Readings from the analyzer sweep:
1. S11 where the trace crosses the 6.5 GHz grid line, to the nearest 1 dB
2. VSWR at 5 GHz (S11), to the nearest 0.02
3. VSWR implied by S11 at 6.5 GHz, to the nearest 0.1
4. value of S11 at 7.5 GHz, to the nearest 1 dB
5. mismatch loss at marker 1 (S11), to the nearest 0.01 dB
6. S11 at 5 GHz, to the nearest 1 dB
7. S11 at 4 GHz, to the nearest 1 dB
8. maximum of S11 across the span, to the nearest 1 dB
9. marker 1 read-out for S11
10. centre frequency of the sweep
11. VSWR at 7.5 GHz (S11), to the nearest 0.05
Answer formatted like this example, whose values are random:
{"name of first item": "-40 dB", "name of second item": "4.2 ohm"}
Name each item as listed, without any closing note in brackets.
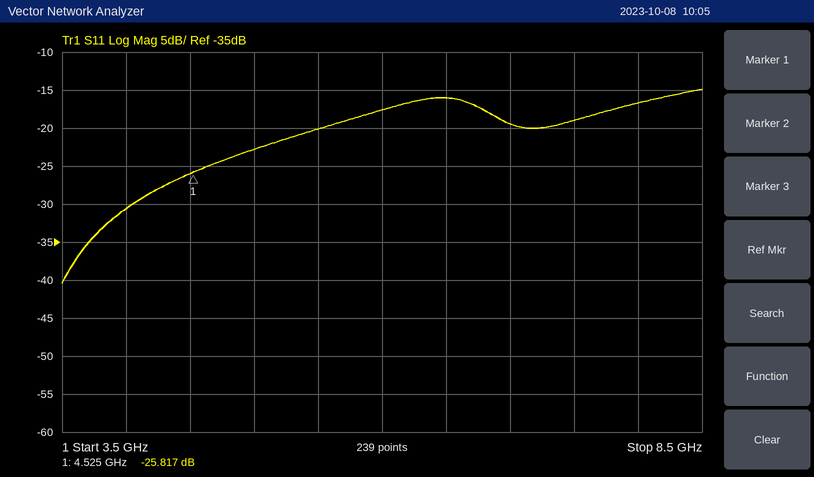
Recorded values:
{"S11 where the trace crosses the 6.5 GHz grid line, to the nearest 1 dB": "-16 dB", "VSWR at 5 GHz (S11), to the nearest 0.02": "1.16", "VSWR implied by S11 at 6.5 GHz, to the nearest 0.1": "1.4", "value of S11 at 7.5 GHz, to the nearest 1 dB": "-19 dB", "mismatch loss at marker 1 (S11), to the nearest 0.01 dB": "0.01 dB", "S11 at 5 GHz, to the nearest 1 dB": "-23 dB", "S11 at 4 GHz, to the nearest 1 dB": "-31 dB", "maximum of S11 across the span, to the nearest 1 dB": "-15 dB", "marker 1 read-out for S11": "-25.817 dB", "centre frequency of the sweep": "6 GHz", "VSWR at 7.5 GHz (S11), to the nearest 0.05": "1.25"}
